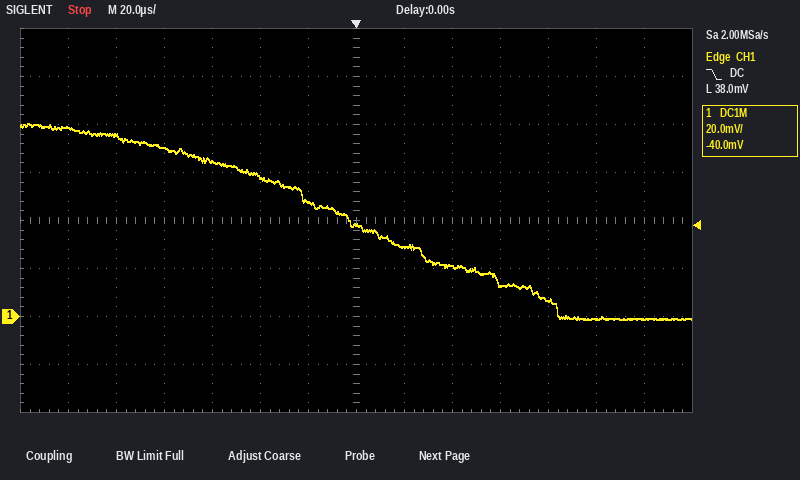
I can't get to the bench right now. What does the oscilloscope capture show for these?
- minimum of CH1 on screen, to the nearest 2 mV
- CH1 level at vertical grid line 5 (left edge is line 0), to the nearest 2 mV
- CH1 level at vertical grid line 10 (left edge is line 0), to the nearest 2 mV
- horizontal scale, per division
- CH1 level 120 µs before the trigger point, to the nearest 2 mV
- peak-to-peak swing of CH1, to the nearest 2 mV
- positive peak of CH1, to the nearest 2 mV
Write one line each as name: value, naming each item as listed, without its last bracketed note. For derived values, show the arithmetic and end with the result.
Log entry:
minimum of CH1 on screen, to the nearest 2 mV: -2 mV
CH1 level at vertical grid line 5 (left edge is line 0), to the nearest 2 mV: 58 mV
CH1 level at vertical grid line 10 (left edge is line 0), to the nearest 2 mV: 14 mV
horizontal scale, per division: 20 µs
CH1 level 120 µs before the trigger point, to the nearest 2 mV: 78 mV
peak-to-peak swing of CH1, to the nearest 2 mV: 80 mV − (-2 mV) = 82 mV
positive peak of CH1, to the nearest 2 mV: 80 mV
